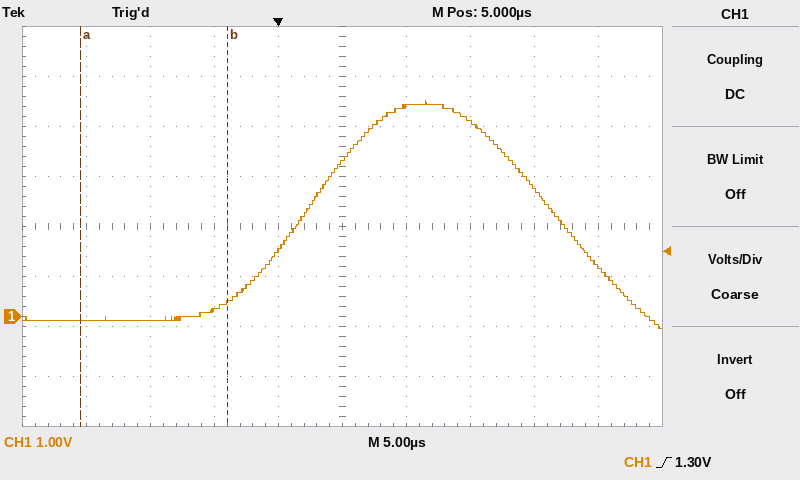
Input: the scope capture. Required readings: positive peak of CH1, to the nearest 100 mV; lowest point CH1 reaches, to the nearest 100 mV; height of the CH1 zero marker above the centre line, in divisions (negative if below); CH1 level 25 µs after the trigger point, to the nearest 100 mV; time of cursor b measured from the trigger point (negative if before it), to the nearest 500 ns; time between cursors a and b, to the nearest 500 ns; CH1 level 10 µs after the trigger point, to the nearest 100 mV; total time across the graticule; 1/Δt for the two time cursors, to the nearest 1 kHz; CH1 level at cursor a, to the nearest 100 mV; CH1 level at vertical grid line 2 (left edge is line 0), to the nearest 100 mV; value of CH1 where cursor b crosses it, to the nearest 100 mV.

4.3 V
-200 mV
-1.8 div
1.0 V
-4.0 µs
11.5 µs
4.2 V
50 µs
87 kHz
-100 mV
-100 mV
300 mV
